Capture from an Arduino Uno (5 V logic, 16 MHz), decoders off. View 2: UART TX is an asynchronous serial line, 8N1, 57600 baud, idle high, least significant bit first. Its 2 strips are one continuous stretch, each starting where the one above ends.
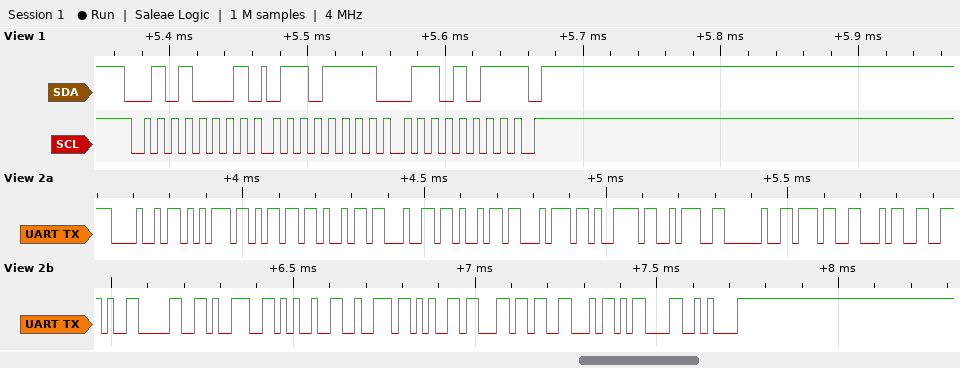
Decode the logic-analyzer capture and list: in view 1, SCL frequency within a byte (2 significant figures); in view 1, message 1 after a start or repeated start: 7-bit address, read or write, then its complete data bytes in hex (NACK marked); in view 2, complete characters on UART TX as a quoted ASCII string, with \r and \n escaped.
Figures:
100 kHz
0x28 read: 6F 6B NACK
"Humidity: 74.09%relF\r\n"
